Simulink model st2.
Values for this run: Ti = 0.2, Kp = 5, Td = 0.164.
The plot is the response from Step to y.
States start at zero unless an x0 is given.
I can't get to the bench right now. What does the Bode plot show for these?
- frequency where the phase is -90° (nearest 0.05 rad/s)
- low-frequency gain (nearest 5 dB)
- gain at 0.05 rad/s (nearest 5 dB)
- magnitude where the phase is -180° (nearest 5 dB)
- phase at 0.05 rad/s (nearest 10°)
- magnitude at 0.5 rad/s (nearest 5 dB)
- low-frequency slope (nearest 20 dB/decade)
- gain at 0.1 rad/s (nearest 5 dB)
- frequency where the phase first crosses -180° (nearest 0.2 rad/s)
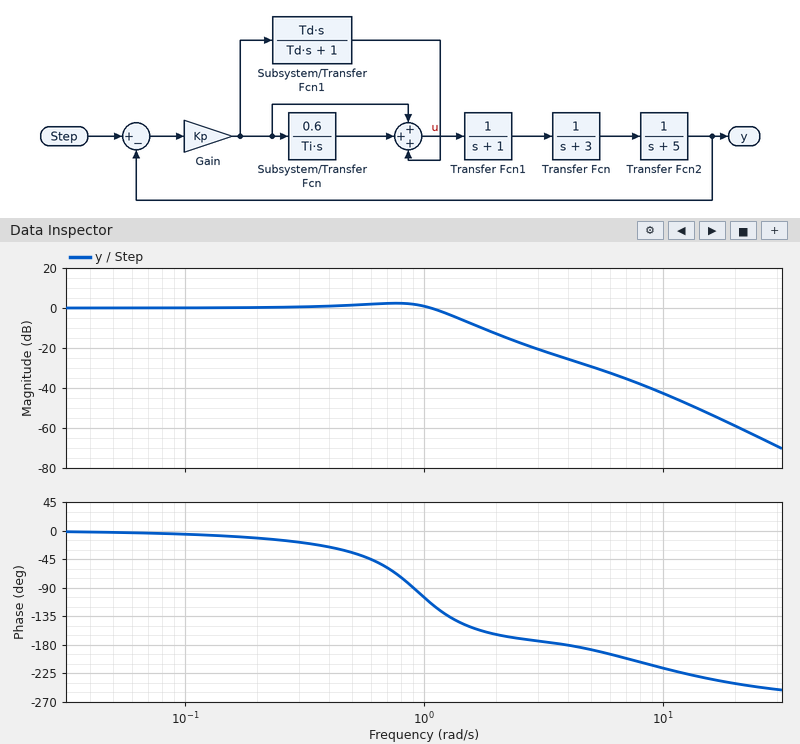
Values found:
0.90 rad/s
0 dB
0 dB
-25 dB
0°
0 dB
0 dB/decade
0 dB
4.0 rad/s
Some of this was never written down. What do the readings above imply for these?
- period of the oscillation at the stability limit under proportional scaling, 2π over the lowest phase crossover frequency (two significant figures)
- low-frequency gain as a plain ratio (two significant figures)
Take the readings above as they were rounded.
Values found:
1.6 s
1.0
